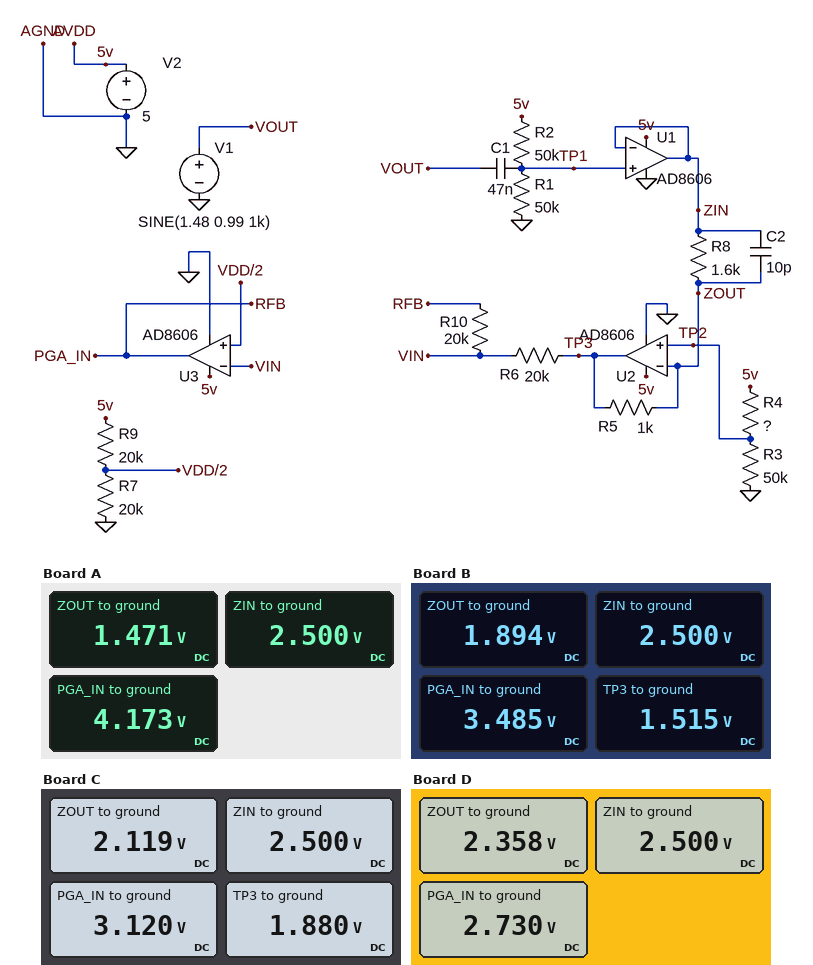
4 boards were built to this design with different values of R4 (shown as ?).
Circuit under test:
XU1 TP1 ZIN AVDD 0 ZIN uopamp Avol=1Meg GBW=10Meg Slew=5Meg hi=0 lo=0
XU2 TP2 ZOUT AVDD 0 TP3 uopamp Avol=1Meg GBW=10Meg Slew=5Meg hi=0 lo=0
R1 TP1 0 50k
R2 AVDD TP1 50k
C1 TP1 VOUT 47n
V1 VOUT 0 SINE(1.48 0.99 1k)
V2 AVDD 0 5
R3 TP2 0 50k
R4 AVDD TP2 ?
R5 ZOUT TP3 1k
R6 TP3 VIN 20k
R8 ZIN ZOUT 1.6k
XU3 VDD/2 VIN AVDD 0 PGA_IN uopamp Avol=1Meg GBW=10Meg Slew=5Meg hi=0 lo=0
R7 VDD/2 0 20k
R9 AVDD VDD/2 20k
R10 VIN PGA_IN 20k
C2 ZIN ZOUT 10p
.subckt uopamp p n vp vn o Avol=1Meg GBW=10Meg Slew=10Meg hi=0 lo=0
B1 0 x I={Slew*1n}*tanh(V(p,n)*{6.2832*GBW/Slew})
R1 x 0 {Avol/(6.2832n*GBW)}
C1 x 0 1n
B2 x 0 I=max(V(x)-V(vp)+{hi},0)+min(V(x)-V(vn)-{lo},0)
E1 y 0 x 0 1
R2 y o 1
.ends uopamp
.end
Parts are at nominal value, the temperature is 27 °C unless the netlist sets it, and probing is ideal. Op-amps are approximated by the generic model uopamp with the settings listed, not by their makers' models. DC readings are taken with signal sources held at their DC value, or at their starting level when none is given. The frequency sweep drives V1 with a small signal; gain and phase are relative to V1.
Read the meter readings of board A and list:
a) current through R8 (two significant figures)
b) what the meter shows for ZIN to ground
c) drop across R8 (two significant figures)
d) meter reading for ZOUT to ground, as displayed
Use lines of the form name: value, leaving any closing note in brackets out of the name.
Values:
current through R8: 640 µA
what the meter shows for ZIN to ground: 2.500 V
drop across R8: 1.0 V
meter reading for ZOUT to ground, as displayed: 1.471 V
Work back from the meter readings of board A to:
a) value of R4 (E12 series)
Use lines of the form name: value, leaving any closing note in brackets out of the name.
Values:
value of R4: 120 kΩ
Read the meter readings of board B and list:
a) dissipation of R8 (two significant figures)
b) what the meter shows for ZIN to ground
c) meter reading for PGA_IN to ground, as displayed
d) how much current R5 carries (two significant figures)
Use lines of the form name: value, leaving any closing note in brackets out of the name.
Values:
dissipation of R8: 230 µW
what the meter shows for ZIN to ground: 2.500 V
meter reading for PGA_IN to ground, as displayed: 3.485 V
how much current R5 carries: 380 µA
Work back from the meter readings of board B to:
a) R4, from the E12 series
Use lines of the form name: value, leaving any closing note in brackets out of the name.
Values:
R4, from the E12 series: 82 kΩ
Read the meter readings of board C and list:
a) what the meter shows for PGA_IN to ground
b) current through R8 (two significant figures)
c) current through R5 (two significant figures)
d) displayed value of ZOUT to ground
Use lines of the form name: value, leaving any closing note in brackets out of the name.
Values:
what the meter shows for PGA_IN to ground: 3.120 V
current through R8: 240 µA
current through R5: 240 µA
displayed value of ZOUT to ground: 2.119 V
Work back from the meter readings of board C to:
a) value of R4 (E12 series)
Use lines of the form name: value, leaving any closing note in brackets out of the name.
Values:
value of R4: 68 kΩ
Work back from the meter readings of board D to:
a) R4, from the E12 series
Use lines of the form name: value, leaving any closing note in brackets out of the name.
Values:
R4, from the E12 series: 56 kΩ
